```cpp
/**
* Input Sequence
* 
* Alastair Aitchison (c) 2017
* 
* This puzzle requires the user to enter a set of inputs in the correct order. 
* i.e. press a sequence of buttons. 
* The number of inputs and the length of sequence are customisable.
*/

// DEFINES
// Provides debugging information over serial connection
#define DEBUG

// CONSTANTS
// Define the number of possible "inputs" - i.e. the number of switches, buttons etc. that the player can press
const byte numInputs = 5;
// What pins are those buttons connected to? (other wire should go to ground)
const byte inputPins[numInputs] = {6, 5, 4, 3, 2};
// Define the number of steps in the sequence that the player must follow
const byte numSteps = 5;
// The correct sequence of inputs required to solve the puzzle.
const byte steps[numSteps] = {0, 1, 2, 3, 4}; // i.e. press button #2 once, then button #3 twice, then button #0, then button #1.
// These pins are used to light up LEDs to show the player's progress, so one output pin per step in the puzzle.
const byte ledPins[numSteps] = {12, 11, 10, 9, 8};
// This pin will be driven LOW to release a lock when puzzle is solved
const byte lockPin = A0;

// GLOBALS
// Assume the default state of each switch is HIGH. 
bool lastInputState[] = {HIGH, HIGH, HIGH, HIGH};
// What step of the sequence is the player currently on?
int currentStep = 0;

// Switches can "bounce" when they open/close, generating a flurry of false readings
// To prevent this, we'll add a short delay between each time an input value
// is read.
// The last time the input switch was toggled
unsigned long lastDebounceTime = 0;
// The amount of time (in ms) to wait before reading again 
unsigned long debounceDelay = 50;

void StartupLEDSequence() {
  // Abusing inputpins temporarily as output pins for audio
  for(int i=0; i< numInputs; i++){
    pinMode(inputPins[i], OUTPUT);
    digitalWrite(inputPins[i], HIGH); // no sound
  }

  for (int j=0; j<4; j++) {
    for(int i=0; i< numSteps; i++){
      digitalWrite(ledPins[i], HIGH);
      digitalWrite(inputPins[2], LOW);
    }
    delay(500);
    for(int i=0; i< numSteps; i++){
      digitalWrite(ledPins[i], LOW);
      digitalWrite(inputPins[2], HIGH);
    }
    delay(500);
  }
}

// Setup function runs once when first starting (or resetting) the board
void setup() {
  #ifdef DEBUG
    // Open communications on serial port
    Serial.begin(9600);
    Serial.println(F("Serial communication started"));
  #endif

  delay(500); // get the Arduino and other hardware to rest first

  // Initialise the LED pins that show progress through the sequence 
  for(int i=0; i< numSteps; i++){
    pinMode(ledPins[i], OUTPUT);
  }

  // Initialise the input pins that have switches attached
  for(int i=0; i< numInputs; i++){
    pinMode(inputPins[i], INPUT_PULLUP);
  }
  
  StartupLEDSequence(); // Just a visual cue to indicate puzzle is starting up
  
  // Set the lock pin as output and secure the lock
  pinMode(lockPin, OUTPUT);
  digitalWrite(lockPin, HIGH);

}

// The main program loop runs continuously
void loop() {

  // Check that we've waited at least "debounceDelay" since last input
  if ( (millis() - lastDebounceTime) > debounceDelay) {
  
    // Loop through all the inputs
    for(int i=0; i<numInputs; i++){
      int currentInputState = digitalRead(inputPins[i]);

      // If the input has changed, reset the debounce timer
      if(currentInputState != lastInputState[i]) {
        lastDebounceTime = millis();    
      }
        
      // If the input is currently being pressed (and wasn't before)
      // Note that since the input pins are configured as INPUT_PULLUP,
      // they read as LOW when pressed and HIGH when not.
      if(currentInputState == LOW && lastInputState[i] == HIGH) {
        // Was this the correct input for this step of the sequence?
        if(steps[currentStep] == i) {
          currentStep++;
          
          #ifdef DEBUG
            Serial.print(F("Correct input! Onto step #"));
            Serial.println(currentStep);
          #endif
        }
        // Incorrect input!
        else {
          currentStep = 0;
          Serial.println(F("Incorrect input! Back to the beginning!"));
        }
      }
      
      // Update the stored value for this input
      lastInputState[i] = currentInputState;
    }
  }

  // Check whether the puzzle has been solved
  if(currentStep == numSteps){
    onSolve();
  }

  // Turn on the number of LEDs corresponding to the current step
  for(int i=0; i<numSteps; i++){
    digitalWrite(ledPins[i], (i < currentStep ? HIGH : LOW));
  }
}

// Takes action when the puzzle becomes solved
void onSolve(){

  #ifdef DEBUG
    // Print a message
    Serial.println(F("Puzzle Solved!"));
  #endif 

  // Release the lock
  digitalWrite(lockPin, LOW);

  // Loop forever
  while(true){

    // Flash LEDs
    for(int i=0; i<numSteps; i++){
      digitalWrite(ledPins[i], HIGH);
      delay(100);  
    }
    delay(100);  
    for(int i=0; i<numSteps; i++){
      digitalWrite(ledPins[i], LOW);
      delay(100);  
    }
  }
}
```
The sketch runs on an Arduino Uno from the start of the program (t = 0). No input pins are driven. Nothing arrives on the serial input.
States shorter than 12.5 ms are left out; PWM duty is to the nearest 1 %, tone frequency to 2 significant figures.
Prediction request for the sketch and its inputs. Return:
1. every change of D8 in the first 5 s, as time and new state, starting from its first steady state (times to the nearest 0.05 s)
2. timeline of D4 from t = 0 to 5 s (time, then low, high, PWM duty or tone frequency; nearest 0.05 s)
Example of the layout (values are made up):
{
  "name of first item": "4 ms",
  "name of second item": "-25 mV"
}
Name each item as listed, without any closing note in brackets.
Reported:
{
  "every change of D8 in the first 5 s, as time and new state, starting from its first steady state": "0.5 s high; 1 s low; 1.5 s high; 2 s low; 2.5 s high; 3 s low; 3.5 s high; 4 s low",
  "timeline of D4 from t = 0 to 5 s": "0.5 s low; 1 s high; 1.5 s low; 2 s high; 2.5 s low; 3 s high; 3.5 s low; 4 s high"
}
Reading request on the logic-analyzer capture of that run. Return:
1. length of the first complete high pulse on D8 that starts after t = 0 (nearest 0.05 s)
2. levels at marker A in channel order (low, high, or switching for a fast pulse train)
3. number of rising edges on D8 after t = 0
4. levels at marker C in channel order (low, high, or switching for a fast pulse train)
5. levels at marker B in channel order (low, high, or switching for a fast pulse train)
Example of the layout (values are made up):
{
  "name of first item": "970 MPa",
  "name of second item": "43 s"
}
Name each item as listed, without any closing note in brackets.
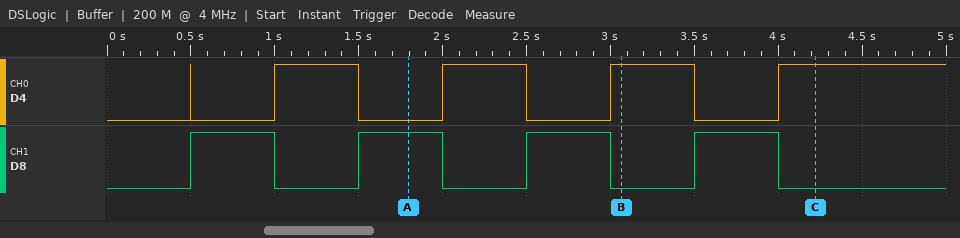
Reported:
{
  "length of the first complete high pulse on D8 that starts after t = 0": "0.50 s",
  "levels at marker A in channel order": "D4 low, D8 high",
  "number of rising edges on D8 after t = 0": "4",
  "levels at marker C in channel order": "D4 high, D8 low",
  "levels at marker B in channel order": "D4 high, D8 low"
}
